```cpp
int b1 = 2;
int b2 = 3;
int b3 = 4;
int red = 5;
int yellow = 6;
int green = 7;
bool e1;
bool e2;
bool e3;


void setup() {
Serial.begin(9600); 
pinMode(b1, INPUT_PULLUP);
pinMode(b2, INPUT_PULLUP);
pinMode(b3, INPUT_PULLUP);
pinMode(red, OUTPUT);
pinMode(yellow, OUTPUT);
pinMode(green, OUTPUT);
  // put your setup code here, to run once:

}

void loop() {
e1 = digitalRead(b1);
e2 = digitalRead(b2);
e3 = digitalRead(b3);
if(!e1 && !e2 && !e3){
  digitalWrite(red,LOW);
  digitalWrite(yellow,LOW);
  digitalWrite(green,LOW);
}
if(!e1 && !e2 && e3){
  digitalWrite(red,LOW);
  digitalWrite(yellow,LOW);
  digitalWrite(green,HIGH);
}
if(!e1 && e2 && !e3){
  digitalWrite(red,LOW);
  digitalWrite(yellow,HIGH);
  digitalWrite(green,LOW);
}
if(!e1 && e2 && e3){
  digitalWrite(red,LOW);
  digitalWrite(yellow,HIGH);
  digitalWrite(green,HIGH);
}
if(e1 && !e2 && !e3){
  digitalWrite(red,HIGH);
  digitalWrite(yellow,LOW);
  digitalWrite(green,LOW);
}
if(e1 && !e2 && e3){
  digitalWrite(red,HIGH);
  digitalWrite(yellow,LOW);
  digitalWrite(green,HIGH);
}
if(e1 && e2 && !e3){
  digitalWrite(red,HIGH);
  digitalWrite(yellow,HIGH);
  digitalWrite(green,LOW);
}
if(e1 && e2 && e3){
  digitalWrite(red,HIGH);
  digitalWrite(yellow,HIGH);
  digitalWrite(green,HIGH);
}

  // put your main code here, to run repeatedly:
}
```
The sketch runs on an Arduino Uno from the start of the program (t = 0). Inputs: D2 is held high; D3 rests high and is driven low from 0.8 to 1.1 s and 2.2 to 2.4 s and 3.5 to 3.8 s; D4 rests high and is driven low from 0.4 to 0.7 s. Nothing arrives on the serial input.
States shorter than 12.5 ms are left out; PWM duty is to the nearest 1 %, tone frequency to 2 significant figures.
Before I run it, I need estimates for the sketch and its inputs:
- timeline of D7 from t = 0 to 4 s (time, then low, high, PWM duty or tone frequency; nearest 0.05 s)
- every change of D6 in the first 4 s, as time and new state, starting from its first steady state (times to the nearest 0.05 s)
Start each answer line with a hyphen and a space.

- 0 s high; 0.4 s low; 0.7 s high
- 0 s high; 0.8 s low; 1.1 s high; 2.2 s low; 2.4 s high; 3.5 s low; 3.8 s high
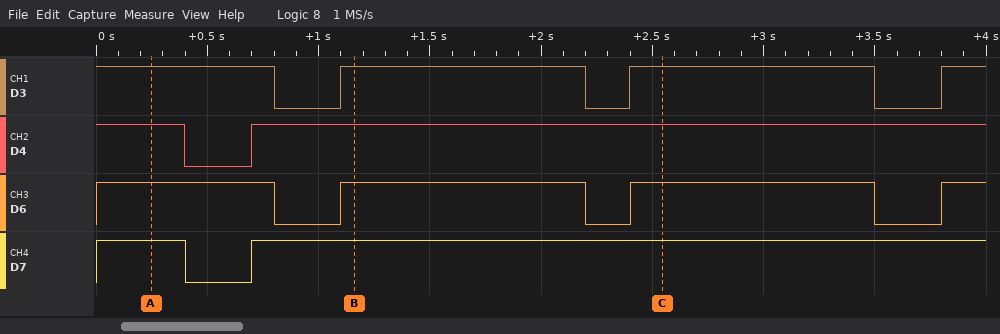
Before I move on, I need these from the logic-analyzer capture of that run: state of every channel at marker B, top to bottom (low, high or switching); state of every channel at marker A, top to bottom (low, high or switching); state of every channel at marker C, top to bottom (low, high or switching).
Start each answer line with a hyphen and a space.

- D3 high, D4 high, D6 high, D7 high
- D3 high, D4 high, D6 high, D7 high
- D3 high, D4 high, D6 high, D7 high
